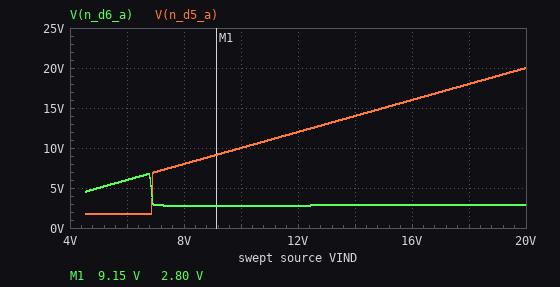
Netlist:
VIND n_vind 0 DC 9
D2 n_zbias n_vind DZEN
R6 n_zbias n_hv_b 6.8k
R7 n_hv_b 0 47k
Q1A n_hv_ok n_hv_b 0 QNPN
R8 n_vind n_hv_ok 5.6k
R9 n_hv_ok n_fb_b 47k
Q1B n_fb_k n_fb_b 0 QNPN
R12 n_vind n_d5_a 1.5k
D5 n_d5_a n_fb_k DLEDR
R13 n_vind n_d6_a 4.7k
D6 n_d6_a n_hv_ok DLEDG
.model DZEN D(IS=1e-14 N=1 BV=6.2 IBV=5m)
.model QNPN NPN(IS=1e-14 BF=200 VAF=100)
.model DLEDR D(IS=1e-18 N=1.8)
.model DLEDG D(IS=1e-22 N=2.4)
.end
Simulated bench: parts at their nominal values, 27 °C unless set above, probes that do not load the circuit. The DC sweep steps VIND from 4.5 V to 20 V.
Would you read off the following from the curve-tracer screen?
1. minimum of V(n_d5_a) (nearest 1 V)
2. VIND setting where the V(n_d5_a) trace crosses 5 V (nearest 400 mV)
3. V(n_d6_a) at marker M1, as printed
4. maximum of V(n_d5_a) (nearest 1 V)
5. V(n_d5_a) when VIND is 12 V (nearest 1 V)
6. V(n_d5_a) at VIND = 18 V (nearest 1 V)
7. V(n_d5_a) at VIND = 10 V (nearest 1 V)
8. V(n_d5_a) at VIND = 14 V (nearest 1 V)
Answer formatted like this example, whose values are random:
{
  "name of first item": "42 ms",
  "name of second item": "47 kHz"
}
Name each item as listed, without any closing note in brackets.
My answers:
{
  "minimum of V(n_d5_a)": "2 V",
  "VIND setting where the V(n_d5_a) trace crosses 5 V": "6.8 V",
  "V(n_d6_a) at marker M1, as printed": "2.80 V",
  "maximum of V(n_d5_a)": "20 V",
  "V(n_d5_a) when VIND is 12 V": "12 V",
  "V(n_d5_a) at VIND = 18 V": "18 V",
  "V(n_d5_a) at VIND = 10 V": "10 V",
  "V(n_d5_a) at VIND = 14 V": "14 V"
}
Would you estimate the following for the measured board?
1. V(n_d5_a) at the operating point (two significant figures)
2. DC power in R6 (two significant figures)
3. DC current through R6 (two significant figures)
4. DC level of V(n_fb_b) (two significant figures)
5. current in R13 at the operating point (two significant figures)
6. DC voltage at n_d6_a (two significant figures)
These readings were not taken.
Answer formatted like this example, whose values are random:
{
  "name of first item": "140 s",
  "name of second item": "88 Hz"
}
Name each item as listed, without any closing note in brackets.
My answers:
{
  "V(n_d5_a) at the operating point": "9.0 V",
  "DC power in R6": "700 µW",
  "DC current through R6": "320 µA",
  "DC level of V(n_fb_b)": "65 mV",
  "current in R13 at the operating point": "1.3 mA",
  "DC voltage at n_d6_a": "2.8 V"
}
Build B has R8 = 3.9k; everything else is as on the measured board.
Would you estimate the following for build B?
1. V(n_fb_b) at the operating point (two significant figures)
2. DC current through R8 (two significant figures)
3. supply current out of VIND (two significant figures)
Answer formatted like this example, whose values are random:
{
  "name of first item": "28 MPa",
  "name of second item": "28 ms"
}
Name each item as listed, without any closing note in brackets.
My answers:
{
  "V(n_fb_b) at the operating point": "70 mV",
  "DC current through R8": "2.3 mA",
  "supply current out of VIND": "3.9 mA"
}
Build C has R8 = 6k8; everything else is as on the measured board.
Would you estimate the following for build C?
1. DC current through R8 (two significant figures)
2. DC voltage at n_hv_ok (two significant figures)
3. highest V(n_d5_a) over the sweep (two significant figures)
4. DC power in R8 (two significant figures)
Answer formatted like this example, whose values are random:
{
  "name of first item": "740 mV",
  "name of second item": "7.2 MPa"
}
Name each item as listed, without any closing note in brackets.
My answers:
{
  "DC current through R8": "1.3 mA",
  "DC voltage at n_hv_ok": "62 mV",
  "highest V(n_d5_a) over the sweep": "20 V",
  "DC power in R8": "12 mW"
}
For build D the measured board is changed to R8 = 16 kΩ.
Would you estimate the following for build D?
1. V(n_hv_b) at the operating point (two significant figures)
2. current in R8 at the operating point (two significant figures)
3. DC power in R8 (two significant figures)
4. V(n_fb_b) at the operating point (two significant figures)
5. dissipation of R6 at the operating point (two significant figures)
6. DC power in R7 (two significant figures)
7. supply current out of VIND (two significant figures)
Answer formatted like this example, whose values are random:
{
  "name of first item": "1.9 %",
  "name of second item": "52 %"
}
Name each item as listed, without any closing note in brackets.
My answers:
{
  "V(n_hv_b) at the operating point": "680 mV",
  "current in R8 at the operating point": "560 µA",
  "DC power in R8": "5.0 mW",
  "V(n_fb_b) at the operating point": "55 mV",
  "dissipation of R6 at the operating point": "710 µW",
  "DC power in R7": "9.8 µW",
  "supply current out of VIND": "2.2 mA"
}
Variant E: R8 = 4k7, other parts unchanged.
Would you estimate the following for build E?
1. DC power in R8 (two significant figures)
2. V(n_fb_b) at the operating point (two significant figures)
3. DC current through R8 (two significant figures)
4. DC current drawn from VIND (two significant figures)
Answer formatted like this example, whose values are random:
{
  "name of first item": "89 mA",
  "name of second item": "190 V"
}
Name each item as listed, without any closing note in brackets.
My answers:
{
  "DC power in R8": "17 mW",
  "V(n_fb_b) at the operating point": "67 mV",
  "DC current through R8": "1.9 mA",
  "DC current drawn from VIND": "3.5 mA"
}
